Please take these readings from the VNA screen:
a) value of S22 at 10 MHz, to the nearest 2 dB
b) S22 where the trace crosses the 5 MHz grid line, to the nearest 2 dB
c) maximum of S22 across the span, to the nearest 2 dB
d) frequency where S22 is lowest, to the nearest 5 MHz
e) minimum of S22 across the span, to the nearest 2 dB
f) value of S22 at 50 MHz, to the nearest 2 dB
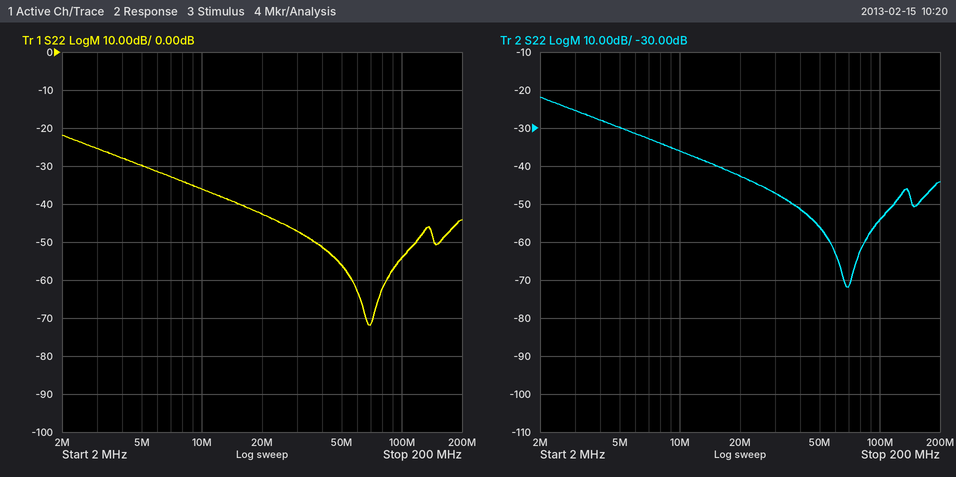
-36 dB
-30 dB
-22 dB
70 MHz
-72 dB
-56 dB
